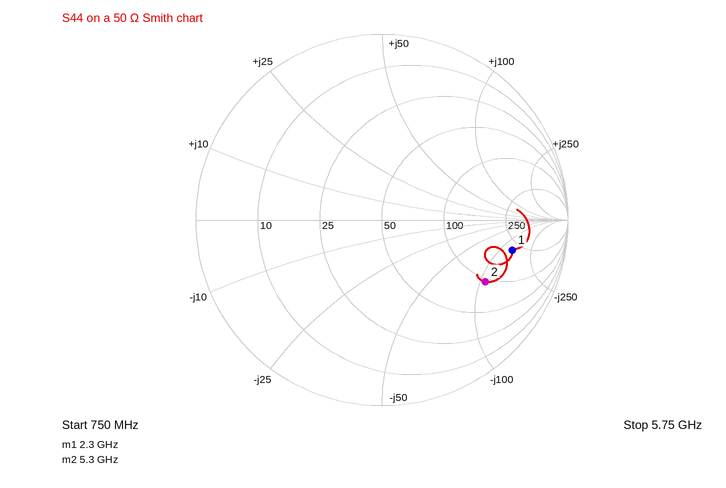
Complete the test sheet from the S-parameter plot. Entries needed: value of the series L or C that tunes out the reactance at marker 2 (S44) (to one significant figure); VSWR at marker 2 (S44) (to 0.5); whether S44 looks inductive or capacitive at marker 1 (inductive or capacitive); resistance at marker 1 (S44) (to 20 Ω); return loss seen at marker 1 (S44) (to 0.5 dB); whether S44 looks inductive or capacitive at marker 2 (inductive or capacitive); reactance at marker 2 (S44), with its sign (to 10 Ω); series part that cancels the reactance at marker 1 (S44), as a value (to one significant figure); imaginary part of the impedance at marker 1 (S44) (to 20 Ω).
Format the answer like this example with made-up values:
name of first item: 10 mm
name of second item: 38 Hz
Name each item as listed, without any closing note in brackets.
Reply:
value of the series L or C that tunes out the reactance at marker 2 (S44): 3 nH
VSWR at marker 2 (S44): 4.5
whether S44 looks inductive or capacitive at marker 1: capacitive
resistance at marker 1 (S44): 200 Ω
return loss seen at marker 1 (S44): 3.0 dB
whether S44 looks inductive or capacitive at marker 2: capacitive
reactance at marker 2 (S44), with its sign: -110 Ω
series part that cancels the reactance at marker 1 (S44), as a value: 10 nH
imaginary part of the impedance at marker 1 (S44): -140 Ω
